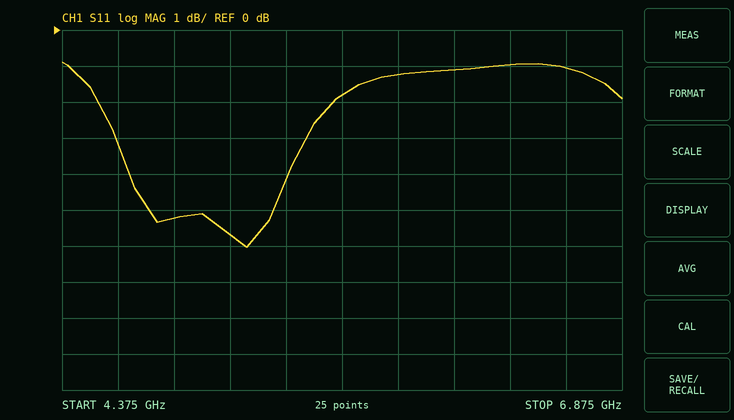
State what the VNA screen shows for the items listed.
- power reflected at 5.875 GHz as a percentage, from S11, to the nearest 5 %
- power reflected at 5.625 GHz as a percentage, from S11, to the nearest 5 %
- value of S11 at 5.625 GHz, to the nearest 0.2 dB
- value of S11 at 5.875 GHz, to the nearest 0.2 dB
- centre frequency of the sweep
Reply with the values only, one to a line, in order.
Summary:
75 %
65 %
-1.8 dB
-1.2 dB
5.625 GHz
